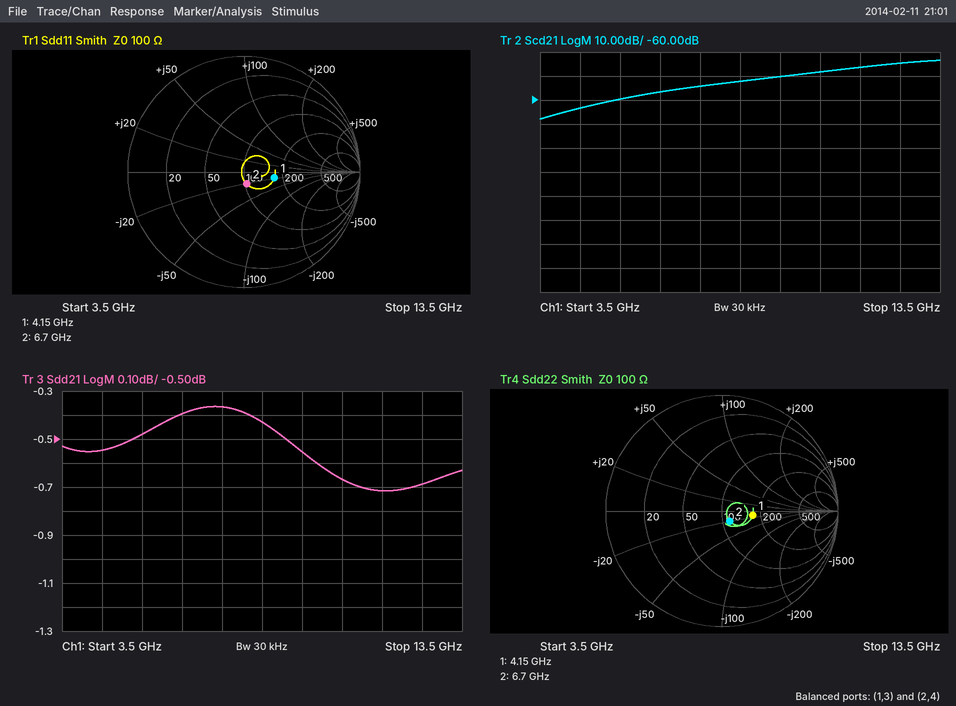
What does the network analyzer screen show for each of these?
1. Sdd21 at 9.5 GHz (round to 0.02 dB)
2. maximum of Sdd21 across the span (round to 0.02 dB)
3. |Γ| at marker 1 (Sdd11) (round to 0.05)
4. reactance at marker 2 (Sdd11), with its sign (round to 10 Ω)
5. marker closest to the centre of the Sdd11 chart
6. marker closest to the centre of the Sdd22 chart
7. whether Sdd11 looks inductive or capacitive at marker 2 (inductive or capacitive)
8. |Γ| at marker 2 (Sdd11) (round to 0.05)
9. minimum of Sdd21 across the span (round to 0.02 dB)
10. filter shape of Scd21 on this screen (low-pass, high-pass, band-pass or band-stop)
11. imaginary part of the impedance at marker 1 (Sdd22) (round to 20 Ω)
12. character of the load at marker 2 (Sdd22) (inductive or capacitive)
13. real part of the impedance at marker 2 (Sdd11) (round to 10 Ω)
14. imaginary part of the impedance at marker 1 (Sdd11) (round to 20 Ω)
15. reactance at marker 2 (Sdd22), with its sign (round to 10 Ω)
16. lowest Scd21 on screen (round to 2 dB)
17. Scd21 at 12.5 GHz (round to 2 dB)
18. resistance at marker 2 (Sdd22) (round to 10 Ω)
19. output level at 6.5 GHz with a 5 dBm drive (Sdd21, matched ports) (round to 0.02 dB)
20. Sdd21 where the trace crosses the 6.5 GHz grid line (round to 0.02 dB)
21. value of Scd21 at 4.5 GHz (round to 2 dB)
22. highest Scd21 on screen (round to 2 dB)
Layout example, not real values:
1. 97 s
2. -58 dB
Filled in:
1. -0.56 dB
2. -0.36 dB
3. 0.25
4. -20 Ω
5. marker 2
6. marker 2
7. capacitive
8. 0.10
9. -0.72 dB
10. high-pass
11. -20 Ω
12. capacitive
13. 100 Ω
14. -20 Ω
15. -20 Ω
16. -68 dB
17. -44 dB
18. 110 Ω
19. 4.60 dBm
20. -0.40 dB
21. -64 dB
22. -44 dB
